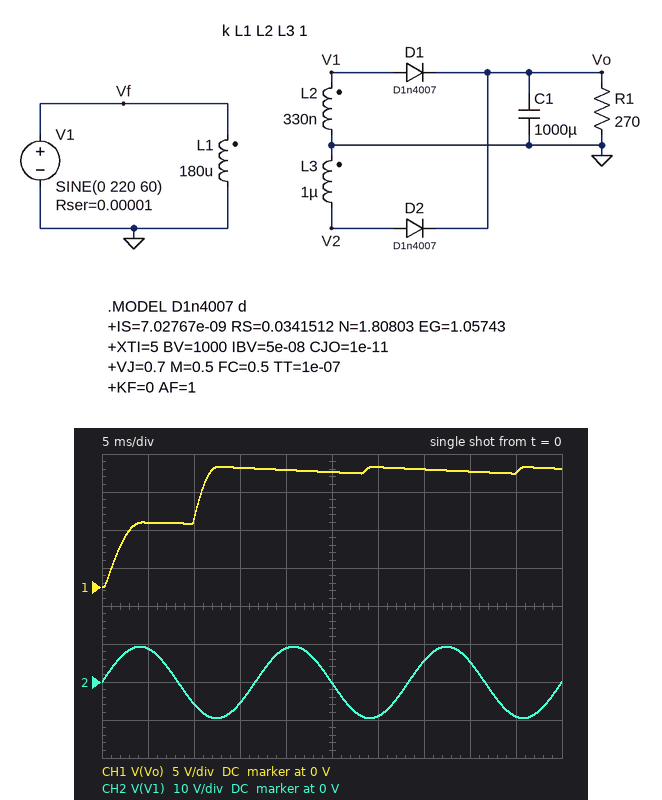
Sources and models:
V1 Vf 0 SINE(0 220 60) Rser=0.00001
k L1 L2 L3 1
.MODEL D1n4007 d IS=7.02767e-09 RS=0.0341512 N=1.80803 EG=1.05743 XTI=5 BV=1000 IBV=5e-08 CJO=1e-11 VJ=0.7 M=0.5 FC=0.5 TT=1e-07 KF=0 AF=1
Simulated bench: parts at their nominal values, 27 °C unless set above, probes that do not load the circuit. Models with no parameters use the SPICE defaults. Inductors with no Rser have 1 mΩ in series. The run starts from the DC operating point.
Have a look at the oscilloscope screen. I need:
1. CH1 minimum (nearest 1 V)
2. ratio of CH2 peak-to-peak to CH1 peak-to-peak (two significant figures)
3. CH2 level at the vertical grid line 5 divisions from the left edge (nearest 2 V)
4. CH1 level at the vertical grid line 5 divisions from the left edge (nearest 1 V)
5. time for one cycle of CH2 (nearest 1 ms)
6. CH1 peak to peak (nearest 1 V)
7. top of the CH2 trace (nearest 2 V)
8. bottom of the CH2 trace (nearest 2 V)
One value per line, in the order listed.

0 V
1.2
0 V
15 V
17 ms
16 V
10 V
-10 V
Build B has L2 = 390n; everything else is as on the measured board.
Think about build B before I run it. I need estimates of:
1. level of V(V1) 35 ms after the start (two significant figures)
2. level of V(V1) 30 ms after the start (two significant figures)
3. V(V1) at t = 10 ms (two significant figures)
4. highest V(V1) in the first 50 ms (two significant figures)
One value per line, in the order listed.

6.0 V
-9.8 V
-6.3 V
10 V
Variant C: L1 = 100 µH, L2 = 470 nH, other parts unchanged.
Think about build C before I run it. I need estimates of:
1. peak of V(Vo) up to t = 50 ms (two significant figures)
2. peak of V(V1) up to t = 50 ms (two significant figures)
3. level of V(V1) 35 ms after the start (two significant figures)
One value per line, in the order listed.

22 V
15 V
8.9 V
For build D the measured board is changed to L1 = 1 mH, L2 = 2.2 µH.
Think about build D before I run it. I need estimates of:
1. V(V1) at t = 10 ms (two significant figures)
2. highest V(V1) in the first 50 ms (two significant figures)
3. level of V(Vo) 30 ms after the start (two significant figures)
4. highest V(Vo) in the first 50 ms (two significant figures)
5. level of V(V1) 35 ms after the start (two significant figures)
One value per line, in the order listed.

-6.1 V
10 V
9.2 V
9.5 V
6.1 V
